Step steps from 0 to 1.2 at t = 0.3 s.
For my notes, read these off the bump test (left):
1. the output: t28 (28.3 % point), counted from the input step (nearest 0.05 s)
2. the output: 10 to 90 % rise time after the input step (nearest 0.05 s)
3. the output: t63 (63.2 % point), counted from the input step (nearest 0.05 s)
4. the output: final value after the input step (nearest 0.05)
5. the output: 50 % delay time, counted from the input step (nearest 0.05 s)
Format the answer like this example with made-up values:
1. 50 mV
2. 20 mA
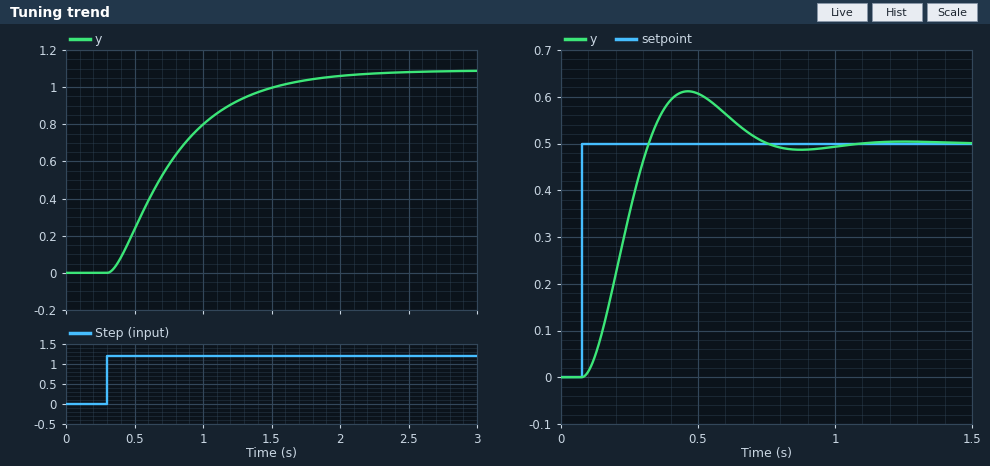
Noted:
1. 0.25 s
2. 1.00 s
3. 0.55 s
4. 1.10
5. 0.40 s
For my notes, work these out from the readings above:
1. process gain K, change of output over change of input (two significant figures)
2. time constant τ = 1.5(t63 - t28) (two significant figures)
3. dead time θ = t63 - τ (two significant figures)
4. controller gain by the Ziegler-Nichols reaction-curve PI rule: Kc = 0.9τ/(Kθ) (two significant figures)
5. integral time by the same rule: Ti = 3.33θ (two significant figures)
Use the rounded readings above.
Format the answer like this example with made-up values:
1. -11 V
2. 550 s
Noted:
1. 0.92
2. 0.45 s
3. 0.10 s
4. 4.4
5. 0.33 s
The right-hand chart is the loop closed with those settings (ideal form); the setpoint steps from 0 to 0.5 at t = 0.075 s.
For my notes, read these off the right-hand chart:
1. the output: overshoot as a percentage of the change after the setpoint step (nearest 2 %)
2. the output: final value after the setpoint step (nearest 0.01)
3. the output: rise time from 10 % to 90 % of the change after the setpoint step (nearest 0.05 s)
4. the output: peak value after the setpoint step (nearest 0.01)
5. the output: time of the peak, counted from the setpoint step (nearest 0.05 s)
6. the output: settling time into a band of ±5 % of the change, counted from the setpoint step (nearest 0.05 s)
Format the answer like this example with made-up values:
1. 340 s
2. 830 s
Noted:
1. 22 %
2. 0.50
3. 0.15 s
4. 0.61
5. 0.40 s
6. 0.60 s
